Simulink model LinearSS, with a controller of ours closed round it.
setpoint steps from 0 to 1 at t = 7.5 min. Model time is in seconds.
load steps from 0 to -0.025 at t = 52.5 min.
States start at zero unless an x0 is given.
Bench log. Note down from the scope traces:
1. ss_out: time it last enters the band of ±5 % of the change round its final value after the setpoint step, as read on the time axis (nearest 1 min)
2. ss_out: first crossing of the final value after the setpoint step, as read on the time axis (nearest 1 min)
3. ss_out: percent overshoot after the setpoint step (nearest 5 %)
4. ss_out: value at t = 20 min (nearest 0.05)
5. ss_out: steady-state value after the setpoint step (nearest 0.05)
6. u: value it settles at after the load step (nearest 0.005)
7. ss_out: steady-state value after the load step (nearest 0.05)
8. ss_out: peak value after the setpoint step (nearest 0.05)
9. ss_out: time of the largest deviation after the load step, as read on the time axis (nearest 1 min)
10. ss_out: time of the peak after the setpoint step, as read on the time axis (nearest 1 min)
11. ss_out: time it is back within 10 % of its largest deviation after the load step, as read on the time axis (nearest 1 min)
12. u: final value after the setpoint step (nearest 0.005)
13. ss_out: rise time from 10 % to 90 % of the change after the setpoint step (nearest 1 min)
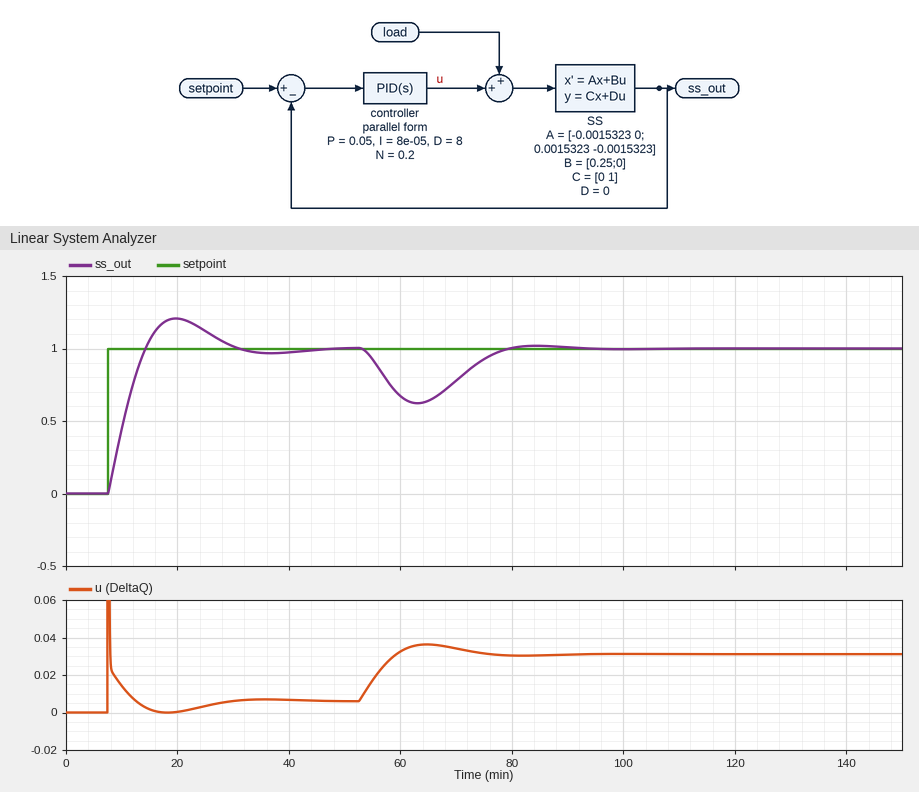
28 min
14 min
20 %
1.20
1.00
0.030
1.00
1.20
63 min
20 min
77 min
0.005
5 min
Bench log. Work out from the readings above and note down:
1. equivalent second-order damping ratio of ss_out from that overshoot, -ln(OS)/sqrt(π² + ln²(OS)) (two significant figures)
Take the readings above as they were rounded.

0.46
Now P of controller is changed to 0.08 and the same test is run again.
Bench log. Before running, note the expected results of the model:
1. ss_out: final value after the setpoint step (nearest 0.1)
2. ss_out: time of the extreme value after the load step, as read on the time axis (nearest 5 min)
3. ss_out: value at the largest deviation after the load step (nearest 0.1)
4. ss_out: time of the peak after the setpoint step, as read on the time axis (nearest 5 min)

1.0
60 min
0.7
15 min
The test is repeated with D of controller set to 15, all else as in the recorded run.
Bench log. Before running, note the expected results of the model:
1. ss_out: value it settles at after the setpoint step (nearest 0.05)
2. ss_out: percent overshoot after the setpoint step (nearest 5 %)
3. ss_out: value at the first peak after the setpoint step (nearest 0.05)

1.00
10 %
1.10
